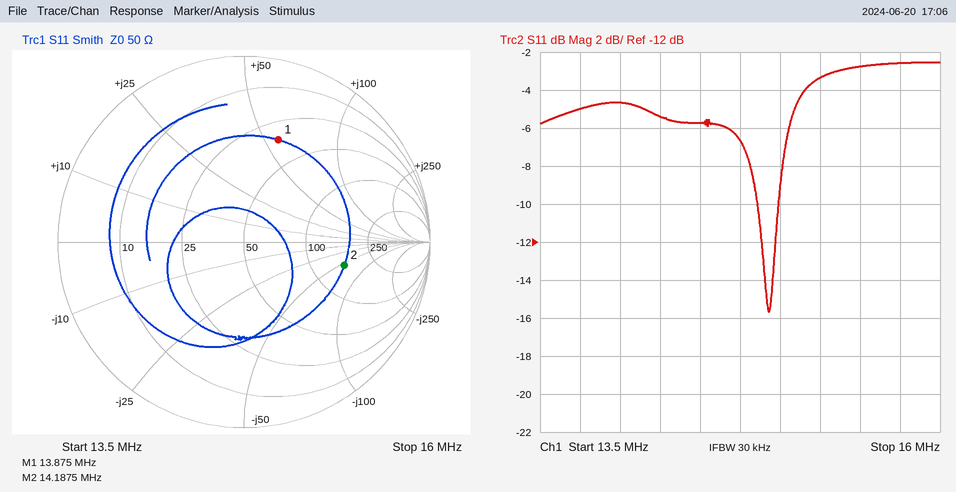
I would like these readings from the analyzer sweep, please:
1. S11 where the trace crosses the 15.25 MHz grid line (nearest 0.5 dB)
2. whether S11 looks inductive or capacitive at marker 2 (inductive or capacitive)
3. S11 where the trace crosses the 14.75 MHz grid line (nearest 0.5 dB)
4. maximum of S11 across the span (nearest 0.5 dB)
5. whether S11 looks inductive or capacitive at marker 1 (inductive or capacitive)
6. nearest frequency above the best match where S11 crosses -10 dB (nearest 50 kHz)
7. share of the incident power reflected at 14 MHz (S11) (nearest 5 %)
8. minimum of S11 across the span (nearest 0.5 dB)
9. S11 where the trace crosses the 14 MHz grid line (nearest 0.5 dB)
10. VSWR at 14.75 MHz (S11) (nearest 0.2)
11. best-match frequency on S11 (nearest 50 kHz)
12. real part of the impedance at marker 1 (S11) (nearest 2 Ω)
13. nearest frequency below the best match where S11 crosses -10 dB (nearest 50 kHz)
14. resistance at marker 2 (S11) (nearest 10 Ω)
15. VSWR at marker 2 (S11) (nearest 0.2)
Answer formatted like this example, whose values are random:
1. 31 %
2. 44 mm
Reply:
1. -3.5 dB
2. capacitive
3. -6.5 dB
4. -2.5 dB
5. inductive
6. 15.00 MHz
7. 35 %
8. -15.5 dB
9. -4.5 dB
10. 2.8
11. 14.95 MHz
12. 34 Ω
13. 14.85 MHz
14. 150 Ω
15. 3.4
